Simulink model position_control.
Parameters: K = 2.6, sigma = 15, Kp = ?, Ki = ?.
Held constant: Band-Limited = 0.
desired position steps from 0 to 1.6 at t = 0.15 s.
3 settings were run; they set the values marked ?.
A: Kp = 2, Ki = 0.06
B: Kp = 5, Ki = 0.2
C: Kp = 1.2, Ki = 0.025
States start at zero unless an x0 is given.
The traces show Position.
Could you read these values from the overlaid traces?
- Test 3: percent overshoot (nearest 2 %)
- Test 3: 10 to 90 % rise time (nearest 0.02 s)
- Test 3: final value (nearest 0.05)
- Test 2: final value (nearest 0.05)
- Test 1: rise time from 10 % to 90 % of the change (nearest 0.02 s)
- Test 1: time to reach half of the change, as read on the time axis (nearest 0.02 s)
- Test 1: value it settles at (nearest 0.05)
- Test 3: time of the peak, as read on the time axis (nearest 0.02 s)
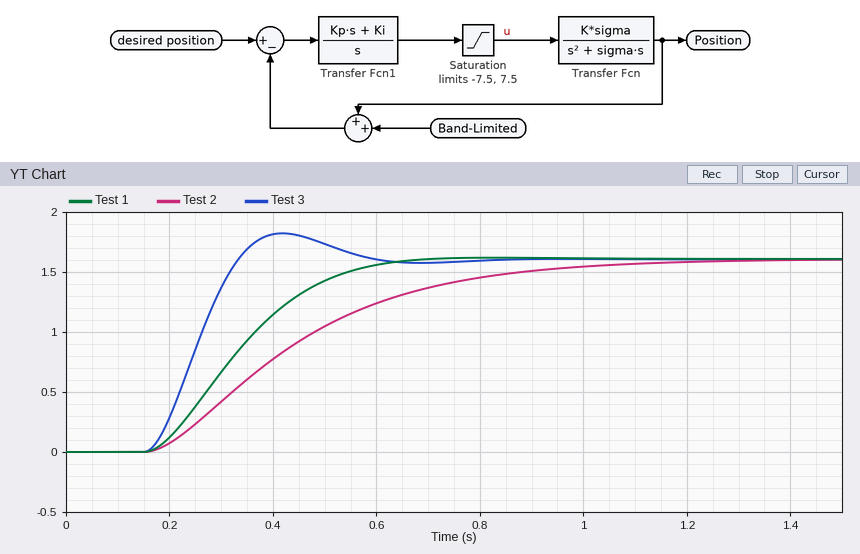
14 %
0.12 s
1.60
1.60
0.30 s
0.32 s
1.60
0.42 s
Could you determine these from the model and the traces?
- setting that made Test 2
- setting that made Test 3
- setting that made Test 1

C
B
A
